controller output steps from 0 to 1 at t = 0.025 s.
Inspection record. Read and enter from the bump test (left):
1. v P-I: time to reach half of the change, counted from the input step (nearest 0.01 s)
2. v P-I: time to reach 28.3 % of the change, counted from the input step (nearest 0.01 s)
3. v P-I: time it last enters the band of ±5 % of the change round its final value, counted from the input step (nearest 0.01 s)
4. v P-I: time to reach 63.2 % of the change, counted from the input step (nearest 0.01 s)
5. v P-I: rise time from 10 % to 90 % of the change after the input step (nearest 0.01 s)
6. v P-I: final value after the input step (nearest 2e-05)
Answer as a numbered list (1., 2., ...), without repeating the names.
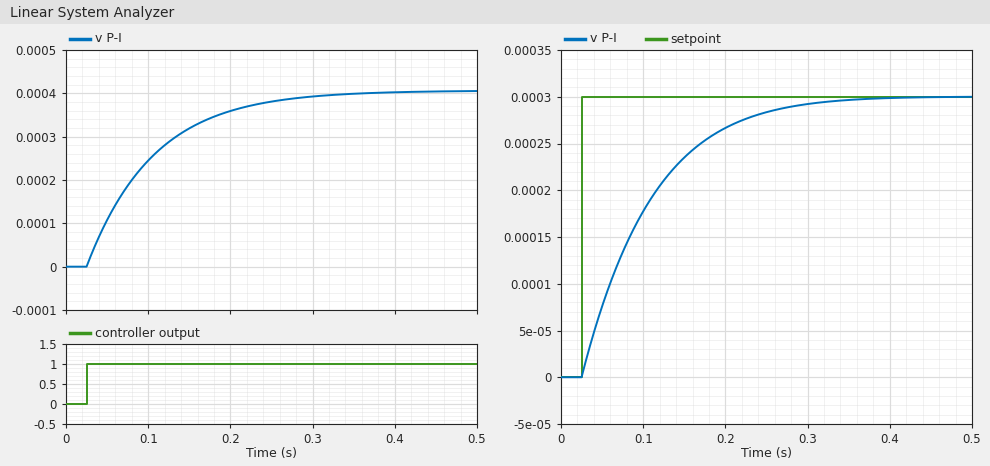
1. 0.06 s
2. 0.03 s
3. 0.24 s
4. 0.08 s
5. 0.18 s
6. 0.00040
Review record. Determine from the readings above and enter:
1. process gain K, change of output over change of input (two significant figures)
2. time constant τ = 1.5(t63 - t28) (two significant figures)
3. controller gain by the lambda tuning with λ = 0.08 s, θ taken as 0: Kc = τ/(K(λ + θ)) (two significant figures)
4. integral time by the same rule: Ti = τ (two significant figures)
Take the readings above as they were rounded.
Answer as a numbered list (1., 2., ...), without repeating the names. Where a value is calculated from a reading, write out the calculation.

1. (0.0004 - 0) / 1 = 0.00040
2. 1.5 × (0.08 - 0.03) = 0.075 s
3. 0.075 / (0.0004 × (0.08 + 0)) = 2300
4. 0.075 s
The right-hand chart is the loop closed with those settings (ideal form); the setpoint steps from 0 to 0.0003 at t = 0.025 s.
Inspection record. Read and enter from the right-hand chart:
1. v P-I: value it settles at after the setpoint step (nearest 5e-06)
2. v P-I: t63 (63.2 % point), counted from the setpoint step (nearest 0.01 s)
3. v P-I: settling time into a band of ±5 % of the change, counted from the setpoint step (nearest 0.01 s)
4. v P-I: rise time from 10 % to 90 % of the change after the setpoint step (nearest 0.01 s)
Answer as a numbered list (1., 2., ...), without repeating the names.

1. 0.000300
2. 0.08 s
3. 0.23 s
4. 0.17 s
